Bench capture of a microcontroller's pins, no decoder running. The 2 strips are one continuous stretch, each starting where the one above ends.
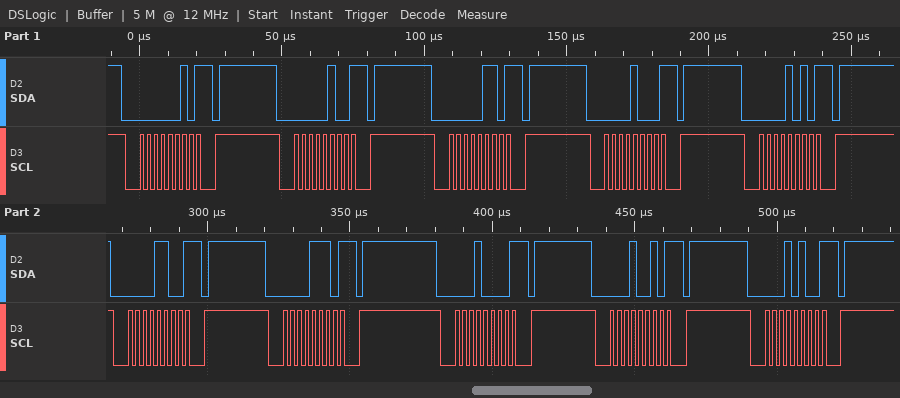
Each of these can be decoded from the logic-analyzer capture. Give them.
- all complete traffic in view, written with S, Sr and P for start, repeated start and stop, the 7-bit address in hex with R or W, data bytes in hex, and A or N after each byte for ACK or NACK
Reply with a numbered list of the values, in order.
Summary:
1. S 01W N P S 02W N P S 03W N P S 04W N P S 05W N P S 06W N P S 07W N P S 08W N P S 09W N P S 0AW N P
